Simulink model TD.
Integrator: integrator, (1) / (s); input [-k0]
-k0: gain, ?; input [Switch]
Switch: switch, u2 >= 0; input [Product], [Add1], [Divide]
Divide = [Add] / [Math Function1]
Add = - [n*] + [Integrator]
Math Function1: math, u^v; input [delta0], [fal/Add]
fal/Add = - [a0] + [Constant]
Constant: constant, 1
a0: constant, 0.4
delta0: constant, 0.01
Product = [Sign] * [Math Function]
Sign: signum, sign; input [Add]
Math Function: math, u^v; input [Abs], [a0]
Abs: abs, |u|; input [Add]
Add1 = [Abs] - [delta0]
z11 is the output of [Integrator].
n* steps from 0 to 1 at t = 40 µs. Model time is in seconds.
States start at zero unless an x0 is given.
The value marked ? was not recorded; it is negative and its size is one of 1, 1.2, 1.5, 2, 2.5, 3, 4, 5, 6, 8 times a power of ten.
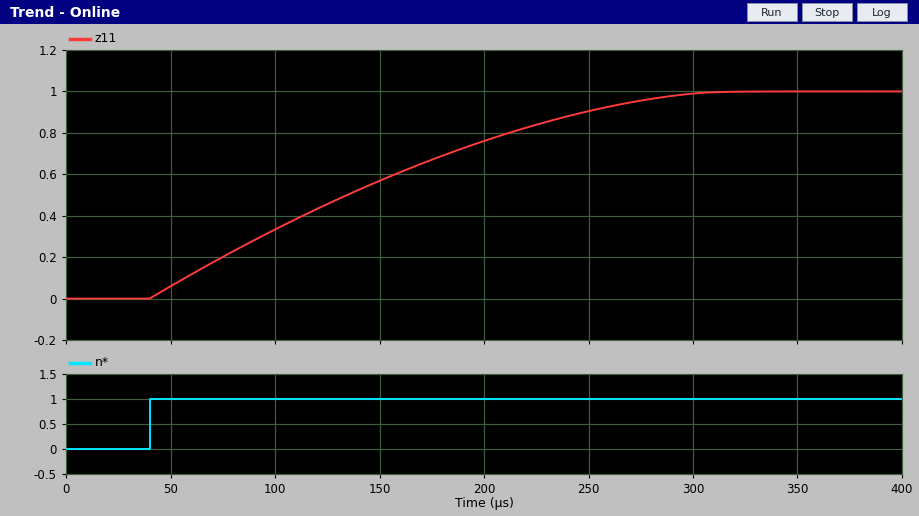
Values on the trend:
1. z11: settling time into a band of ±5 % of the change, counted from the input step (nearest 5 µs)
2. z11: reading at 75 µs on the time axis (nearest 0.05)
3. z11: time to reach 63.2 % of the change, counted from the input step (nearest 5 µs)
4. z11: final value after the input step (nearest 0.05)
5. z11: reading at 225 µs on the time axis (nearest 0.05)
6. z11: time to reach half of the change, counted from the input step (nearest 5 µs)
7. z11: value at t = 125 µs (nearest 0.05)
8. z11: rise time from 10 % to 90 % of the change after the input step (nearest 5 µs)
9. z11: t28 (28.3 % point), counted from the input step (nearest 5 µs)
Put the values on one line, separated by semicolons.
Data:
230 µs; 0.20; 125 µs; 1.00; 0.85; 95 µs; 0.45; 190 µs; 50 µs
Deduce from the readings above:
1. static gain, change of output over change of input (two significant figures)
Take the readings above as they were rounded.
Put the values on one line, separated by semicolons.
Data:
1.0
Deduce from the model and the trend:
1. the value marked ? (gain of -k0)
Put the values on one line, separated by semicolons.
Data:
-6000
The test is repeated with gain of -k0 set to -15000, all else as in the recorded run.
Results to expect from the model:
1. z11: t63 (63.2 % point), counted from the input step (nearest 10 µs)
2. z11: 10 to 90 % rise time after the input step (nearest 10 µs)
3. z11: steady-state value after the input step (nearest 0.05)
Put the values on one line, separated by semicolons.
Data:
50 µs; 80 µs; 1.00
